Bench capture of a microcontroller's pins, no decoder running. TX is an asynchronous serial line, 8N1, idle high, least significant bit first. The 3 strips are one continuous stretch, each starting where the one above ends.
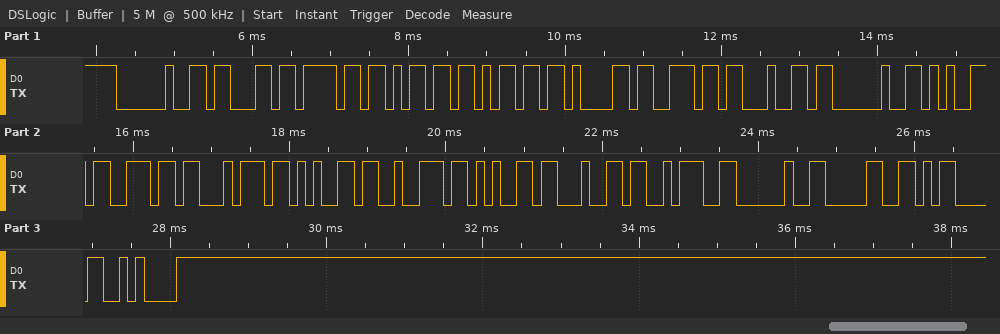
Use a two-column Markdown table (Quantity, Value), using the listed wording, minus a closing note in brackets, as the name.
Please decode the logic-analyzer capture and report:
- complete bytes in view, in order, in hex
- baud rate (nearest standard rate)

| Quantity | Value |
|---|---|
| complete bytes in view, in order, in hex | 20 63 6F 6D 6D 61 6E 64 20 65 6E 74 65 72 65 64 3A 20 30 0D 0A |
| baud rate | 9600 baud |
